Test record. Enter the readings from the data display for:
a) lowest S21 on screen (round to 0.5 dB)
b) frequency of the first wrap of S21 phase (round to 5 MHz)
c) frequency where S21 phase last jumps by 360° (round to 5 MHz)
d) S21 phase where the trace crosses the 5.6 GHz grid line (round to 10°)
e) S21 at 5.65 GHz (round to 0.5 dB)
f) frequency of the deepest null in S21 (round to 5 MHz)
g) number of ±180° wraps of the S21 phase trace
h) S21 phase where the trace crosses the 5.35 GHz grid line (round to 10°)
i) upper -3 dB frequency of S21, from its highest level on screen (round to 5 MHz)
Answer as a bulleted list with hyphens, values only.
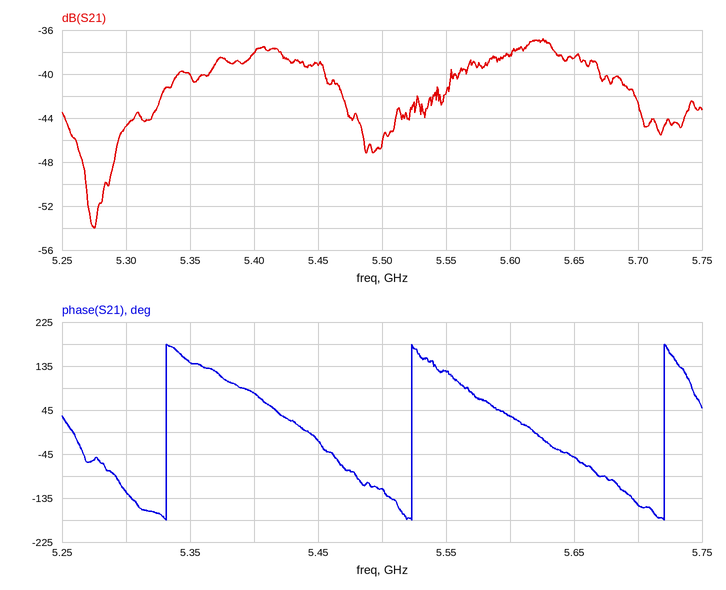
- -54.0 dB
- 5.330 GHz
- 5.720 GHz
- 30°
- -38.5 dB
- 5.275 GHz
- 3
- 140°
- 5.670 GHz
